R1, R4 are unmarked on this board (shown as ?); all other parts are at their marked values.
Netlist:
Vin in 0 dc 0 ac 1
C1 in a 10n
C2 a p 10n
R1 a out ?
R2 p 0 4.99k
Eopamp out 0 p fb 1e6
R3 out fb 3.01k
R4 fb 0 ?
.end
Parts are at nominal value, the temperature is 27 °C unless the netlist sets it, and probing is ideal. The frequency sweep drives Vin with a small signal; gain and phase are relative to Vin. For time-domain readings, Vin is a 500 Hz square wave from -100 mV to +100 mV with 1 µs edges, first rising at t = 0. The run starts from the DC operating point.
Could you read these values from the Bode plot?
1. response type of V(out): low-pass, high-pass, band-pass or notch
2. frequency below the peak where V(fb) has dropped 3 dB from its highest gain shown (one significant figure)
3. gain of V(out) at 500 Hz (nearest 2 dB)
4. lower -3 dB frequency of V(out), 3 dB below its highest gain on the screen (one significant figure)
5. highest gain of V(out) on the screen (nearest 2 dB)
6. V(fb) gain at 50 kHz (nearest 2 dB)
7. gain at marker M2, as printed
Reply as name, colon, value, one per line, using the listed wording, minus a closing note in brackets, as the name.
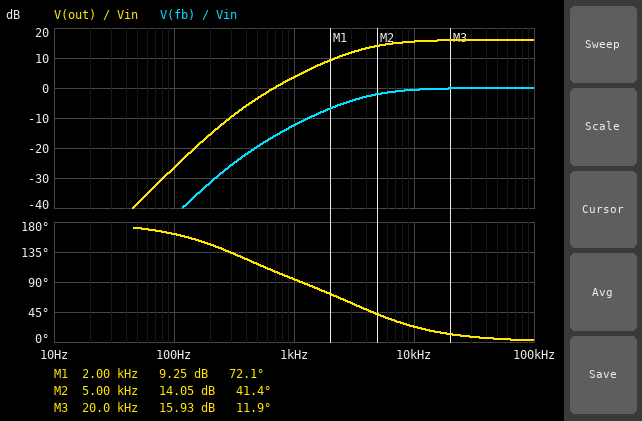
response type of V(out): low-pass, high-pass, band-pass or notch: high-pass
frequency below the peak where V(fb) has dropped 3 dB from its highest gain shown: 4 kHz
gain of V(out) at 500 Hz: -4 dB
lower -3 dB frequency of V(out), 3 dB below its highest gain on the screen: 4 kHz
highest gain of V(out) on the screen: 16 dB
V(fb) gain at 50 kHz: 0 dB
gain at marker M2, as printed: 14.05 dB
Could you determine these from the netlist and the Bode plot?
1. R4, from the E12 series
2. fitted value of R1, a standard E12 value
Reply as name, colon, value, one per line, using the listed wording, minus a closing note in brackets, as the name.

R4, from the E12 series: 560 Ω
fitted value of R1, a standard E12 value: 39 kΩ
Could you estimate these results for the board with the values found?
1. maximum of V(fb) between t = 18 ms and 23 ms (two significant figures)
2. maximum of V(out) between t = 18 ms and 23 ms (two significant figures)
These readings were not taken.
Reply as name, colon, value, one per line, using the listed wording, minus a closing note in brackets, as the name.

maximum of V(fb) between t = 18 ms and 23 ms: 200 mV
maximum of V(out) between t = 18 ms and 23 ms: 1.3 V
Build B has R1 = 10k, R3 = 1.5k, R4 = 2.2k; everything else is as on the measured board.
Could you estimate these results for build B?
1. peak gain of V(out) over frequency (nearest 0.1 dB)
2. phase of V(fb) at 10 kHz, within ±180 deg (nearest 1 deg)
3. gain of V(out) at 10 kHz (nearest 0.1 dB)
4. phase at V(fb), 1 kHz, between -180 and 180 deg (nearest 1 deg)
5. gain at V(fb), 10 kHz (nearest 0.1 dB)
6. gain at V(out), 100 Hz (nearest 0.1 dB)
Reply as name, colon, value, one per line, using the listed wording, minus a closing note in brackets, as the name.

peak gain of V(out) over frequency: 4.5 dB
phase of V(fb) at 10 kHz, within ±180 deg: 29 deg
gain of V(out) at 10 kHz: 3.8 dB
phase at V(fb), 1 kHz, between -180 and 180 deg: 128 deg
gain at V(fb), 10 kHz: -0.7 dB
gain at V(out), 100 Hz: -49.6 dB
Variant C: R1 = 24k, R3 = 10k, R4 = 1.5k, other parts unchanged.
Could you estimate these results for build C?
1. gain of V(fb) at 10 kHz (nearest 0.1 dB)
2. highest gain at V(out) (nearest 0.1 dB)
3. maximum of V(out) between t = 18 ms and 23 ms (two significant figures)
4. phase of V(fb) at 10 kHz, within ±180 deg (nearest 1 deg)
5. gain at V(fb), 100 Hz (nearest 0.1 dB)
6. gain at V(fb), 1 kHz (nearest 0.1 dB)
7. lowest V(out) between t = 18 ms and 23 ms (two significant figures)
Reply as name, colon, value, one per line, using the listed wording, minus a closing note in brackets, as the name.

gain of V(fb) at 10 kHz: 0 dB
highest gain at V(out): 17.7 dB
maximum of V(out) between t = 18 ms and 23 ms: 1.5 V
phase of V(fb) at 10 kHz, within ±180 deg: 11 deg
gain at V(fb), 100 Hz: -46.5 dB
gain at V(fb), 1 kHz: -7.1 dB
lowest V(out) between t = 18 ms and 23 ms: -1.5 V
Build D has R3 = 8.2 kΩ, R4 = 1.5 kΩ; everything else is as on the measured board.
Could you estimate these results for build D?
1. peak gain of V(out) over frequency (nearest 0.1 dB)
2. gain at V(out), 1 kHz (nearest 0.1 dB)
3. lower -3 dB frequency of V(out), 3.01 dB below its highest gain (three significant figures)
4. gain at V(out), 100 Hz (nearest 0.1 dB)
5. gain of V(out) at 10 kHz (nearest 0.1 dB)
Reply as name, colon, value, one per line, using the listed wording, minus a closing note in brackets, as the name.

peak gain of V(out) over frequency: 16.2 dB
gain at V(out), 1 kHz: 3.8 dB
lower -3 dB frequency of V(out), 3.01 dB below its highest gain: 3.84 kHz
gain at V(out), 100 Hz: -26.4 dB
gain of V(out) at 10 kHz: 15.6 dB
